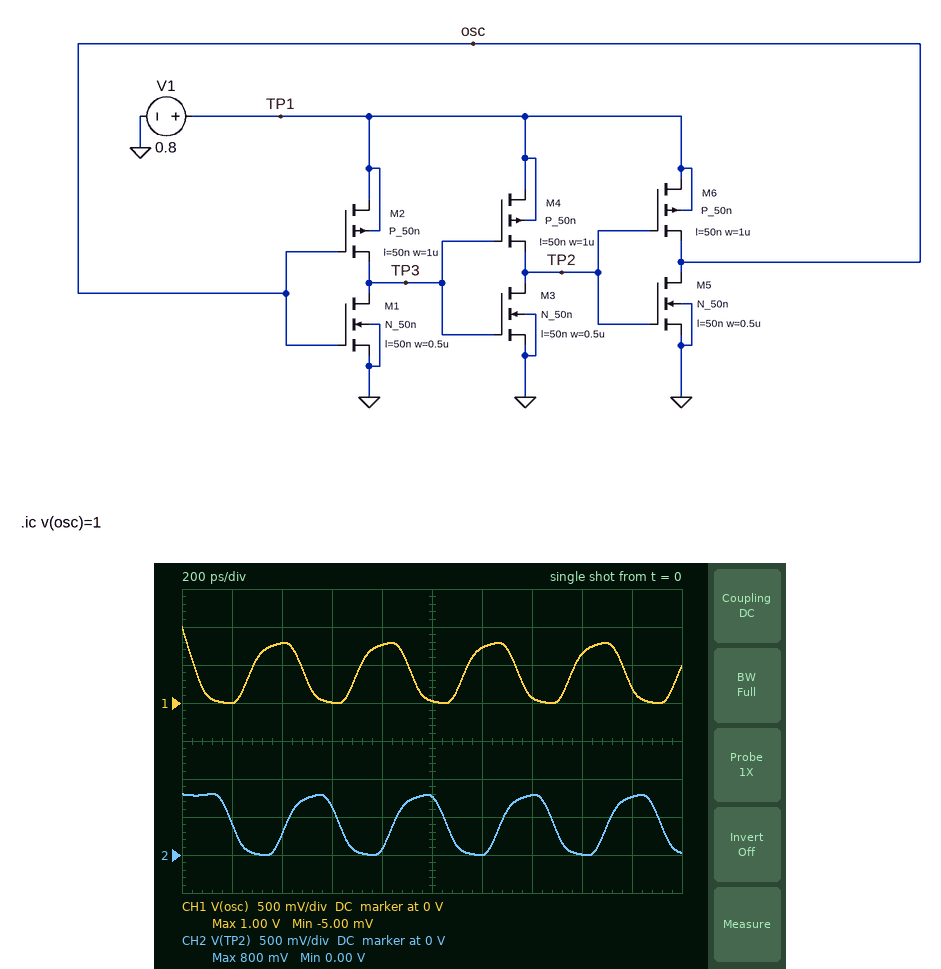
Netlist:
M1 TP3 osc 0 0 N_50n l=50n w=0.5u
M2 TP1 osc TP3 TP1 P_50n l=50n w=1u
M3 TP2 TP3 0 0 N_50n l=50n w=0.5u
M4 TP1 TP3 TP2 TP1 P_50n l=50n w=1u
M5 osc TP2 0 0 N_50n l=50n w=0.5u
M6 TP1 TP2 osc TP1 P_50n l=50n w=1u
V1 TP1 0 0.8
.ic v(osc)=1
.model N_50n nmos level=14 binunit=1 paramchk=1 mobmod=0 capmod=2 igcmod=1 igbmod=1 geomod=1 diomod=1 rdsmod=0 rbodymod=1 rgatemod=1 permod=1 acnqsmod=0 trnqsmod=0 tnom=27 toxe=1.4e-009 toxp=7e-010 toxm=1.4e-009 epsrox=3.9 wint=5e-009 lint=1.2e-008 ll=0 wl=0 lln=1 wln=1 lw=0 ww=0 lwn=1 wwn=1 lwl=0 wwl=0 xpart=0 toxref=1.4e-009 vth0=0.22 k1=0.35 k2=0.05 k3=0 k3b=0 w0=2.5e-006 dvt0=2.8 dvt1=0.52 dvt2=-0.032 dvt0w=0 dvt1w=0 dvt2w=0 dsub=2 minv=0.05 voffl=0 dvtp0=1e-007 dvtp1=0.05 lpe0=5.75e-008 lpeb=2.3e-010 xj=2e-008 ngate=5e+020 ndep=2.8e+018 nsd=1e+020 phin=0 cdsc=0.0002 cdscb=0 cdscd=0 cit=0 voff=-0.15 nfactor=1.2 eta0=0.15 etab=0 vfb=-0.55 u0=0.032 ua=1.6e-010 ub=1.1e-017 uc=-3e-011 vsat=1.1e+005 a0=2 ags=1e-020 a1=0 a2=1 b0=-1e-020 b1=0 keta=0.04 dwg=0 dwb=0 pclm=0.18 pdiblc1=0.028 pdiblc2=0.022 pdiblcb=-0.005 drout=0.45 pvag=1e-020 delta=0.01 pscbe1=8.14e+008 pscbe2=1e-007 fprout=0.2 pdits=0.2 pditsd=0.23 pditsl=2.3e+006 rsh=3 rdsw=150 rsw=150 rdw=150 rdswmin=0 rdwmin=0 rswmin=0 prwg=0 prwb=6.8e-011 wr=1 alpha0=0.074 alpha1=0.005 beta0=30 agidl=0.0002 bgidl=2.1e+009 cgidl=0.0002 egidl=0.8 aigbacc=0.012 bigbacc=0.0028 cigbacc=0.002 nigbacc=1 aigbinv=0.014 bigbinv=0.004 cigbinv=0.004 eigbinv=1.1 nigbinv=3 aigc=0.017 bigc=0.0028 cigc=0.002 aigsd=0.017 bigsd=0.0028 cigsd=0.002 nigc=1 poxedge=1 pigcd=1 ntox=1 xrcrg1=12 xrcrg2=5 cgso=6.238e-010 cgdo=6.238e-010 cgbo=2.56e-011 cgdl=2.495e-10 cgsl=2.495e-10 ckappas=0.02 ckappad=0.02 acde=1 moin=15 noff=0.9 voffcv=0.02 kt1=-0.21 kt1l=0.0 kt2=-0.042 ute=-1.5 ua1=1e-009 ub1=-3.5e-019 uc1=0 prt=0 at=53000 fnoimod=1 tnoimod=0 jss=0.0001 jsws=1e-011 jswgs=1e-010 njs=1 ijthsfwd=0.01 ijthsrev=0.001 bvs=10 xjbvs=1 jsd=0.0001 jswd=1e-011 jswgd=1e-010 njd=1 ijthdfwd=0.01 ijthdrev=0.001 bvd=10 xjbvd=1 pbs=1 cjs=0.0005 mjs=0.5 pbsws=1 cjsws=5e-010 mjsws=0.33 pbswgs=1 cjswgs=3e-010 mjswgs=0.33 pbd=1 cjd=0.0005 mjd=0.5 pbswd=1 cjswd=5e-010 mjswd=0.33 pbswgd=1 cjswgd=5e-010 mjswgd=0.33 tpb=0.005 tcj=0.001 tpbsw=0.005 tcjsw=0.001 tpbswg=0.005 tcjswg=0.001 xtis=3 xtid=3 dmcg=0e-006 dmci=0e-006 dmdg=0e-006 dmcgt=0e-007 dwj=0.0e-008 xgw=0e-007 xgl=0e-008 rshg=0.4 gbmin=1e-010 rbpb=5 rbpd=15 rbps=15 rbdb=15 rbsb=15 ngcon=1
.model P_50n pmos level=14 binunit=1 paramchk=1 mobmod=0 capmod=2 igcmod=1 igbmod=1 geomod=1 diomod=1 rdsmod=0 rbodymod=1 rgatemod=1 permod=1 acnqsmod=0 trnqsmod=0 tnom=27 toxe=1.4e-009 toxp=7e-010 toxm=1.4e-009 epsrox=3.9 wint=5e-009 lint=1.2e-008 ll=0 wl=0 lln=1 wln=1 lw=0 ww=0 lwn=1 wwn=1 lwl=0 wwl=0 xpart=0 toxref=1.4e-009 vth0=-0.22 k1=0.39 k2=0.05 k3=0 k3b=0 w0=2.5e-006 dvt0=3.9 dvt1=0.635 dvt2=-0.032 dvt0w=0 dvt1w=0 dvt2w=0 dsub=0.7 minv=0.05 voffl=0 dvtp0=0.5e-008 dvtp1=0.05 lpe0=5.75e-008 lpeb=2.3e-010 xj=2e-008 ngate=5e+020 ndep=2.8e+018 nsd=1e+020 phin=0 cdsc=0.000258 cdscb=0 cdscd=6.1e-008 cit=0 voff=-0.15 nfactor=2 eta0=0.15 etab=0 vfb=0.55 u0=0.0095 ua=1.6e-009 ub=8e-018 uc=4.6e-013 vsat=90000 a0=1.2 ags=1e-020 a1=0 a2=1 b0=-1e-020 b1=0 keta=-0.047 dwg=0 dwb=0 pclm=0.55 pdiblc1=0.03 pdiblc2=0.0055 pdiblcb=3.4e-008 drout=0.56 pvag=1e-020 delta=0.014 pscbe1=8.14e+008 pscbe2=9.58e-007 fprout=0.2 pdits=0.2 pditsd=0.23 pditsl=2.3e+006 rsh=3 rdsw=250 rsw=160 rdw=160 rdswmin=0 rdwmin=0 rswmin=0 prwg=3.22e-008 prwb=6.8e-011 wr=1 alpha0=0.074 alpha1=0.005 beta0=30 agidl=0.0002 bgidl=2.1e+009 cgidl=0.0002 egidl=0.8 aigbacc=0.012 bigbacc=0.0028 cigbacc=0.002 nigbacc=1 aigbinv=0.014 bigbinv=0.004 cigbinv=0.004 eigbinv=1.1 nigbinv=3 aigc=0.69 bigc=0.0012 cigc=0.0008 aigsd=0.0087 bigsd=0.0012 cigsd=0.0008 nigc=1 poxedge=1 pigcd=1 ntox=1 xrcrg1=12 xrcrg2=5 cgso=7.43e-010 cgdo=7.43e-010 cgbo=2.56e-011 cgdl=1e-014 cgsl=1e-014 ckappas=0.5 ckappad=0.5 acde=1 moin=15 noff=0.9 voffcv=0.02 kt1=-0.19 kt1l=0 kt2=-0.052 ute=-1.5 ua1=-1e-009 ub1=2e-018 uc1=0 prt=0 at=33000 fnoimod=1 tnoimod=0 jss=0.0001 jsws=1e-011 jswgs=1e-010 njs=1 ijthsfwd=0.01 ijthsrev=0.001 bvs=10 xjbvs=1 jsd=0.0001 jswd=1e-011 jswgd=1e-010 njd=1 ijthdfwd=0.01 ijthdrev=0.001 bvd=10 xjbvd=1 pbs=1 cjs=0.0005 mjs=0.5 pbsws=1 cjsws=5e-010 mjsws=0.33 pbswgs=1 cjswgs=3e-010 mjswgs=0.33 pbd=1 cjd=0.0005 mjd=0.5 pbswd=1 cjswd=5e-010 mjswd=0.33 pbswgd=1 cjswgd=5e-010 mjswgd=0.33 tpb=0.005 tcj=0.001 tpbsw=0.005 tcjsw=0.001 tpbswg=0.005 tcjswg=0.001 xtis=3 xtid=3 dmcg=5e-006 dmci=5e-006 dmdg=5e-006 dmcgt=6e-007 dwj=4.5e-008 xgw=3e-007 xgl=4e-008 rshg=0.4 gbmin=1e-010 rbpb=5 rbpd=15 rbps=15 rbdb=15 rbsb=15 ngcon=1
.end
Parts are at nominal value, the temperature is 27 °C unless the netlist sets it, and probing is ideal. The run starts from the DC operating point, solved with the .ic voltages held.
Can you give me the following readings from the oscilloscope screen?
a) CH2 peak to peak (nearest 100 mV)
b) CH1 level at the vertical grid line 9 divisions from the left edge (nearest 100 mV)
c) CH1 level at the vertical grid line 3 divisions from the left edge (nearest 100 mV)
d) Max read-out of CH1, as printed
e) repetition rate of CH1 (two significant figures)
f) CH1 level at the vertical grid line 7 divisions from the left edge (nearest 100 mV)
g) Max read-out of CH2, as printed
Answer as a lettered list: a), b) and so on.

a) 800 mV
b) 200 mV
c) 0 V
d) 1.00 V
e) 2.3 GHz
f) 100 mV
g) 800 mV
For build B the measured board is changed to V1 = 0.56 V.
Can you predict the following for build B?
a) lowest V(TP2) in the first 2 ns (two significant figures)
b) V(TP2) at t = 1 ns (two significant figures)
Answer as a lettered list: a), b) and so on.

a) -7.5 mV
b) 440 mV
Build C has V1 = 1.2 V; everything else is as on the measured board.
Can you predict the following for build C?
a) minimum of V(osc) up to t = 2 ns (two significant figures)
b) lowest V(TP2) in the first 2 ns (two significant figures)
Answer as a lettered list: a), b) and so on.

a) 15 mV
b) 20 mV
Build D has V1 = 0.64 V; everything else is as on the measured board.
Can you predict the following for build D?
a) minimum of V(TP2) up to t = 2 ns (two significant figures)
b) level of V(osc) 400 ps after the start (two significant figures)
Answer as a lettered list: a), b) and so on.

a) -6.2 mV
b) 150 mV
